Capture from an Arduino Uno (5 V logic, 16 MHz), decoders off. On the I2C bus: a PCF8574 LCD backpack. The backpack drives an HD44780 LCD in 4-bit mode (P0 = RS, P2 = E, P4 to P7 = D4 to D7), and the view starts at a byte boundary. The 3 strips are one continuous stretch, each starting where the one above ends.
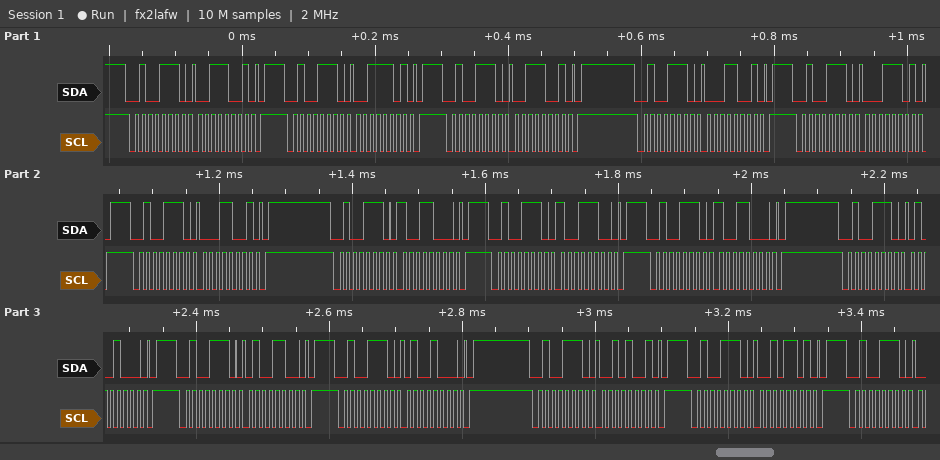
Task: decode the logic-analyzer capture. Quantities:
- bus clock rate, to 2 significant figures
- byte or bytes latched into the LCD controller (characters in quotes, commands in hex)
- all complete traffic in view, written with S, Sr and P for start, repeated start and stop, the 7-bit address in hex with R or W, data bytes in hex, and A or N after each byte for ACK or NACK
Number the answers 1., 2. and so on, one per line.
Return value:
1. 100 kHz
2. '1' 0x94
3. S 27W A 39 A P S 27W A 3D A P S 27W A 39 A P S 27W A 19 A P S 27W A 1D A P S 27W A 19 A P S 27W A 98 A P S 27W A 9C A P S 27W A 98 A P S 27W A 48 A P S 27W A 4C A P S 27W A 48 A P S 27W A 29 A P S 27W A 2D A P S 27W A
